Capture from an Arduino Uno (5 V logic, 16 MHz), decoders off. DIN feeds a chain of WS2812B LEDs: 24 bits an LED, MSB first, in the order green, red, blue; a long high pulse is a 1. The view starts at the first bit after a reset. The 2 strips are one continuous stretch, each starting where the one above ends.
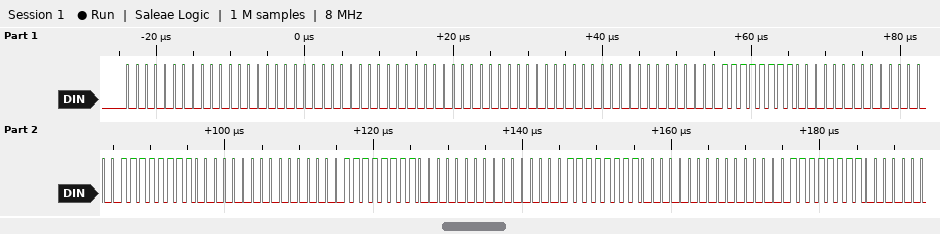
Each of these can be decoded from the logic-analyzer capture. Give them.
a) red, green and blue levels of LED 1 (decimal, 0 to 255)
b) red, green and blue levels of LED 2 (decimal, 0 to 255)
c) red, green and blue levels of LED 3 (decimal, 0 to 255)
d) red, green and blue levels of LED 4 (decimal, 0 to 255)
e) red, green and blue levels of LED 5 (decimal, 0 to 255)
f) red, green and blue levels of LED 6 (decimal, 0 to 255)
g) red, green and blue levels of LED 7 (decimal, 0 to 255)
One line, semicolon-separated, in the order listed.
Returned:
0, 0, 0; 0, 0, 0; 0, 0, 255; 0, 0, 255; 0, 0, 255; 0, 0, 255; 0, 0, 255
